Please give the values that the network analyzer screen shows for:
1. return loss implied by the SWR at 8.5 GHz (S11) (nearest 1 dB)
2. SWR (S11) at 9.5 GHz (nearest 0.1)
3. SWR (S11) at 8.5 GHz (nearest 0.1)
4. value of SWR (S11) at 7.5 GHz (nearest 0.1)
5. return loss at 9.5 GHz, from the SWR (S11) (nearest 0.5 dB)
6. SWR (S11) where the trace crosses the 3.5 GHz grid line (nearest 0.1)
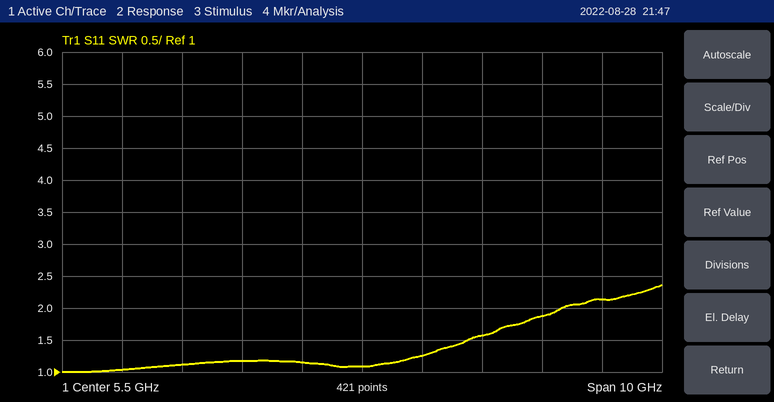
10 dB
2.1
1.9
1.6
9.0 dB
1.2
